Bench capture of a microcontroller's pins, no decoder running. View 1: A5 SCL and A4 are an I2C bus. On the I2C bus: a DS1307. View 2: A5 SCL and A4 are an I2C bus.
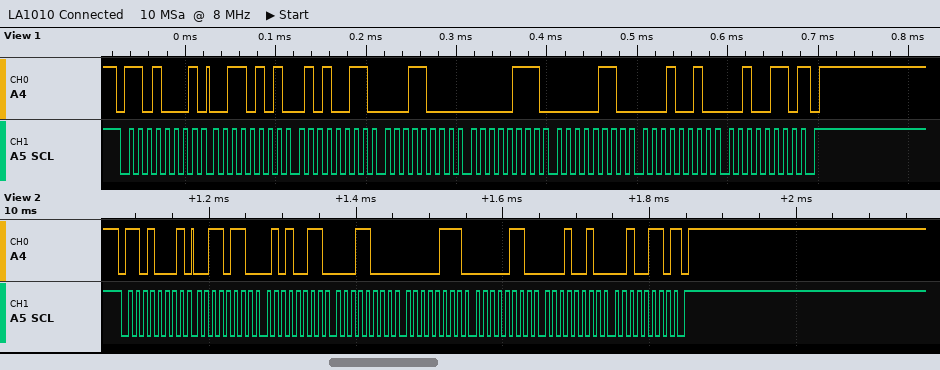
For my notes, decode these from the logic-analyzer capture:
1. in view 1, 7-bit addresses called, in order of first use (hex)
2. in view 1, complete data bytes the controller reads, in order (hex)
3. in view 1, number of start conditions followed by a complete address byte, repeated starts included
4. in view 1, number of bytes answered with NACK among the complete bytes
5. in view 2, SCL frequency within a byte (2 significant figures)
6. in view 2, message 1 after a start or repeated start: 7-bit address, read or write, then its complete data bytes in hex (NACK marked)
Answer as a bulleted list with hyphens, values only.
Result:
- 0x68
- 35 53 18 07 06 12 26
- 1
- 1
- 100 kHz
- 0x68 read: 36 53 18 07 06 12 26 NACK
